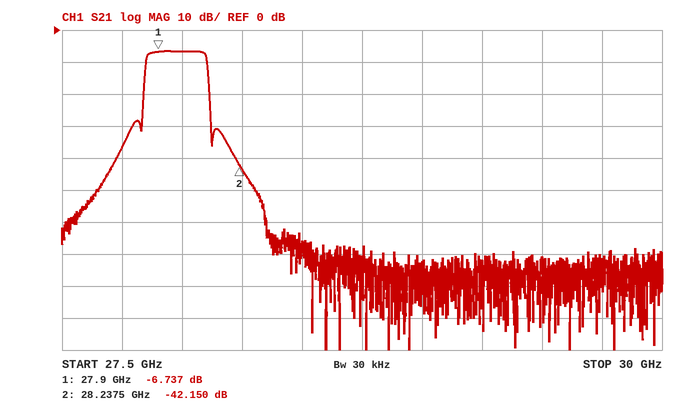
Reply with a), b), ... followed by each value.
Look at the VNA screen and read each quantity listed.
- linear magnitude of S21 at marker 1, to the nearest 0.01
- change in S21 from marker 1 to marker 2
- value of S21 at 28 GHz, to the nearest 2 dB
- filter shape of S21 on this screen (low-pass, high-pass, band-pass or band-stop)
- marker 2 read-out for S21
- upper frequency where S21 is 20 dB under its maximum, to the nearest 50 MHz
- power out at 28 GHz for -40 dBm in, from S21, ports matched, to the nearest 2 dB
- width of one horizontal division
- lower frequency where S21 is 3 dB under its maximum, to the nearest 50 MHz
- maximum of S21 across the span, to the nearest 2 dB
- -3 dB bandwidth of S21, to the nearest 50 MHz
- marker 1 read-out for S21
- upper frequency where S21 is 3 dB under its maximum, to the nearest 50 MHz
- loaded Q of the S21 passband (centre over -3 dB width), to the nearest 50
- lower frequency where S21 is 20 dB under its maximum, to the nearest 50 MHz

a) 0.46
b) -35.413 dB
c) -6 dB
d) band-pass
e) -42.150 dB
f) 28.10 GHz
g) -46 dBm
h) 250 MHz
i) 27.85 GHz
j) -6 dB
k) 250 MHz
l) -6.737 dB
m) 28.10 GHz
n) 100
o) 27.85 GHz
